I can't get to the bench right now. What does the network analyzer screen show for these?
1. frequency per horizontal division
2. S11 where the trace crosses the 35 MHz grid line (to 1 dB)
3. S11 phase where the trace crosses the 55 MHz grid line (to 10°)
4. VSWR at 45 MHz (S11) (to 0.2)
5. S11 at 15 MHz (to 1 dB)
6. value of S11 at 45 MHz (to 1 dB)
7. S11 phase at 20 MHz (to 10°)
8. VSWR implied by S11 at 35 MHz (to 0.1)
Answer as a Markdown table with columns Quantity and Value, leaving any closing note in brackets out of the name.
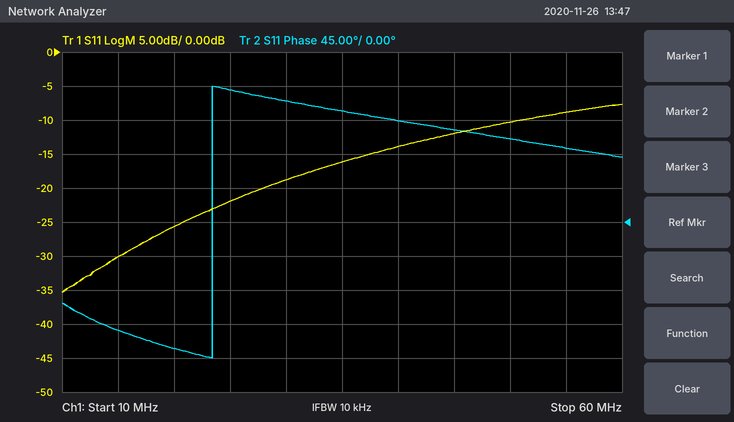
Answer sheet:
| Quantity | Value |
|---|---|
| frequency per horizontal division | 5 MHz |
| S11 where the trace crosses the 35 MHz grid line | -16 dB |
| S11 phase where the trace crosses the 55 MHz grid line | 100° |
| VSWR at 45 MHz (S11) | 1.6 |
| S11 at 15 MHz | -30 dB |
| value of S11 at 45 MHz | -12 dB |
| S11 phase at 20 MHz | -170° |
| VSWR implied by S11 at 35 MHz | 1.4 |
